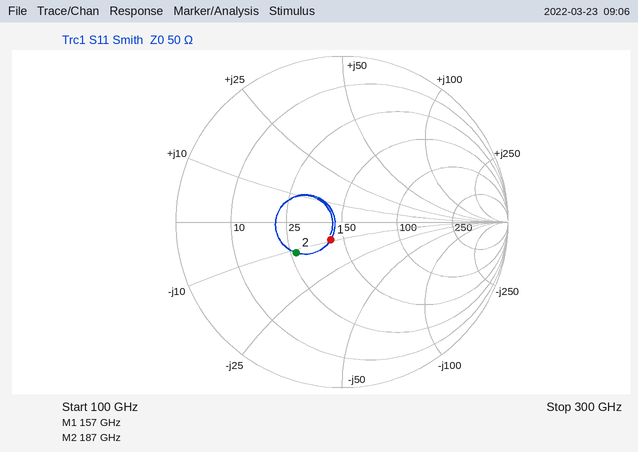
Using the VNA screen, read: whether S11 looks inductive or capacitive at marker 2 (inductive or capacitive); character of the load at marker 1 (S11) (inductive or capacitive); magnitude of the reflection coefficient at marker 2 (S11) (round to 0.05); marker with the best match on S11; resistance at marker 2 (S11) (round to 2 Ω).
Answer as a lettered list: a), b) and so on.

a) capacitive
b) capacitive
c) 0.35
d) marker 1
e) 26 Ω
